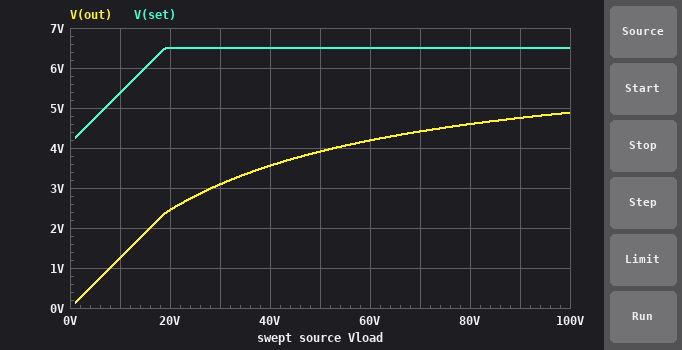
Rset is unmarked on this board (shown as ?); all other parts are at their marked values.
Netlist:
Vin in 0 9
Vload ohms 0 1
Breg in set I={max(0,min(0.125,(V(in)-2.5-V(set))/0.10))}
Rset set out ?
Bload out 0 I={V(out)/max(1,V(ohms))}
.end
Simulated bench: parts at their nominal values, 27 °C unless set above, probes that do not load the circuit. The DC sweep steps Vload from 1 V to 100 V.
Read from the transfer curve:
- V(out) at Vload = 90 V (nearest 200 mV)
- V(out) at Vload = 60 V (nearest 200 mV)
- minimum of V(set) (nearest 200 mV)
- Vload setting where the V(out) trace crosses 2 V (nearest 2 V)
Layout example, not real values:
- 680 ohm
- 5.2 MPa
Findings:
- 4.8 V
- 4.2 V
- 4.2 V
- 16 V
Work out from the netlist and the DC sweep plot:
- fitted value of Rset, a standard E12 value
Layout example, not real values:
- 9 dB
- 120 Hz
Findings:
- 33 Ω
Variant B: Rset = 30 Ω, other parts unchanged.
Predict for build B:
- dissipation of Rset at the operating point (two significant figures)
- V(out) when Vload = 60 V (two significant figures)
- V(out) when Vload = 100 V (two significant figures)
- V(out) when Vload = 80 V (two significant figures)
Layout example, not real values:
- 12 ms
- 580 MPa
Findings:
- 470 mW
- 4.3 V
- 5.0 V
- 4.7 V
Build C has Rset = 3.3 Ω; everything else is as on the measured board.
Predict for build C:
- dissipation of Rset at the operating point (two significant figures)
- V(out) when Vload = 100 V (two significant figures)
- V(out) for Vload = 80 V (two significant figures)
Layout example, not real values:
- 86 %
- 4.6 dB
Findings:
- 52 mW
- 6.3 V
- 6.2 V
